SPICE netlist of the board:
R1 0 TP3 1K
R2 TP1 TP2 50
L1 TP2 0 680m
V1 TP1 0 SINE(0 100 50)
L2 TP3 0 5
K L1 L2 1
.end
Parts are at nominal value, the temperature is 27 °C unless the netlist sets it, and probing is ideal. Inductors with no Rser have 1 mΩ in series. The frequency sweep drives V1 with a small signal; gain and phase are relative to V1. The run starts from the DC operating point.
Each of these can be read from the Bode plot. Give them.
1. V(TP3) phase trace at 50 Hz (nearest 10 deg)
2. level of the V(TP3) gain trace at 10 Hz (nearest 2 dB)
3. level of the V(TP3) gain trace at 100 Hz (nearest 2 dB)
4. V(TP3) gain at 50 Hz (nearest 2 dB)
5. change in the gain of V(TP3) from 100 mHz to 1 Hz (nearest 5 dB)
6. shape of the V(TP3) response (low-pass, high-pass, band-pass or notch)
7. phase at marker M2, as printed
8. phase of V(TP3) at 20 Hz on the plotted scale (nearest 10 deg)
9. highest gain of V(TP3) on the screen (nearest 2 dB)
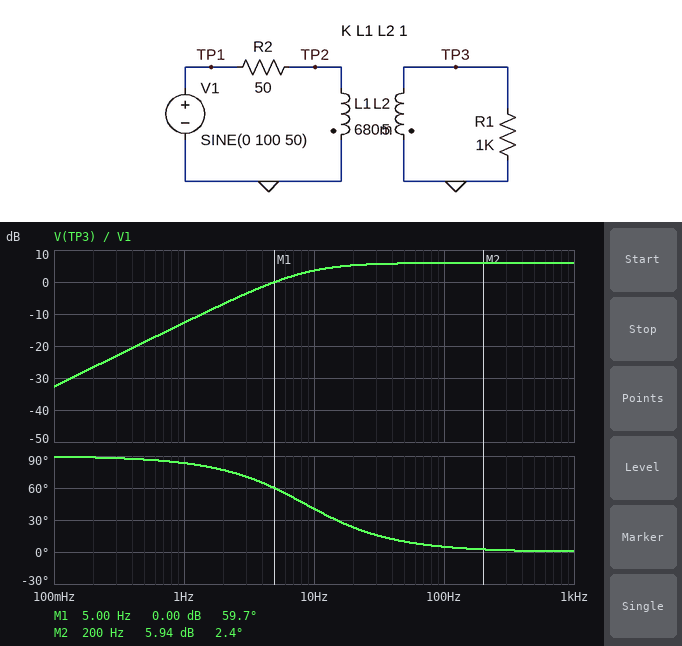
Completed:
10 deg
4 dB
6 dB
6 dB
20 dB
high-pass
2.4 deg
20 deg
6 dB
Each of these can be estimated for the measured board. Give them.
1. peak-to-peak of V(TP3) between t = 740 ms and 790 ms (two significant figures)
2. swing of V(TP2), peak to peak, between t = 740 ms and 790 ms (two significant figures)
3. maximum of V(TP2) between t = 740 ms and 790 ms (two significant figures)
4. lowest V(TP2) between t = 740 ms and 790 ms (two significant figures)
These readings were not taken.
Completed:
390 V
140 V
72 V
-72 V
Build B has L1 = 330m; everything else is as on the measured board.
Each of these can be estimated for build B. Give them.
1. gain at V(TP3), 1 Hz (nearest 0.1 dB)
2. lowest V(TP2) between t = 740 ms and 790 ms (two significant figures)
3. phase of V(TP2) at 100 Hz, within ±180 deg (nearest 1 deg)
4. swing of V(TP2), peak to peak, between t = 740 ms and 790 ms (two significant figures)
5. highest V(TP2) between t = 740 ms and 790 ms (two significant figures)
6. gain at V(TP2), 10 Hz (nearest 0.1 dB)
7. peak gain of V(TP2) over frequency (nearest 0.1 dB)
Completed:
-15.9 dB
-55 V
8 deg
110 V
55 V
-9.5 dB
-4.9 dB
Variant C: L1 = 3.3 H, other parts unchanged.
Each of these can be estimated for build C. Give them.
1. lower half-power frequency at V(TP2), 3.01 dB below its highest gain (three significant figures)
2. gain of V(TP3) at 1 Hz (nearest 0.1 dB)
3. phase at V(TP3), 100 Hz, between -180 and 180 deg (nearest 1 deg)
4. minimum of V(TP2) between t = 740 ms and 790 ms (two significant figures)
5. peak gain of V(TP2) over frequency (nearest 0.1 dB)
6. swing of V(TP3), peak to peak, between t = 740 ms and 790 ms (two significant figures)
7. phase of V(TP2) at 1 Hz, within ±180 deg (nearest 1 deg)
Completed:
2.24 Hz
-6.6 dB
1 deg
-93 V
-0.6 dB
230 V
66 deg
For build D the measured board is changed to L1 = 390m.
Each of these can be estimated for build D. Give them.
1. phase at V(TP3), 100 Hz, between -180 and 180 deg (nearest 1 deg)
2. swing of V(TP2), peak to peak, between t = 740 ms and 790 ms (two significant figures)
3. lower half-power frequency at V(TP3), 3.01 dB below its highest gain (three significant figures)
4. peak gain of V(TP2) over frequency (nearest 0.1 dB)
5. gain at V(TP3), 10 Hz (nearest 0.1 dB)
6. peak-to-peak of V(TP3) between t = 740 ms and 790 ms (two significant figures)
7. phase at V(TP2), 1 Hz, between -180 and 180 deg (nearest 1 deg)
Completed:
7 deg
120 V
12.4 Hz
-4.3 dB
2.7 dB
420 V
85 deg
